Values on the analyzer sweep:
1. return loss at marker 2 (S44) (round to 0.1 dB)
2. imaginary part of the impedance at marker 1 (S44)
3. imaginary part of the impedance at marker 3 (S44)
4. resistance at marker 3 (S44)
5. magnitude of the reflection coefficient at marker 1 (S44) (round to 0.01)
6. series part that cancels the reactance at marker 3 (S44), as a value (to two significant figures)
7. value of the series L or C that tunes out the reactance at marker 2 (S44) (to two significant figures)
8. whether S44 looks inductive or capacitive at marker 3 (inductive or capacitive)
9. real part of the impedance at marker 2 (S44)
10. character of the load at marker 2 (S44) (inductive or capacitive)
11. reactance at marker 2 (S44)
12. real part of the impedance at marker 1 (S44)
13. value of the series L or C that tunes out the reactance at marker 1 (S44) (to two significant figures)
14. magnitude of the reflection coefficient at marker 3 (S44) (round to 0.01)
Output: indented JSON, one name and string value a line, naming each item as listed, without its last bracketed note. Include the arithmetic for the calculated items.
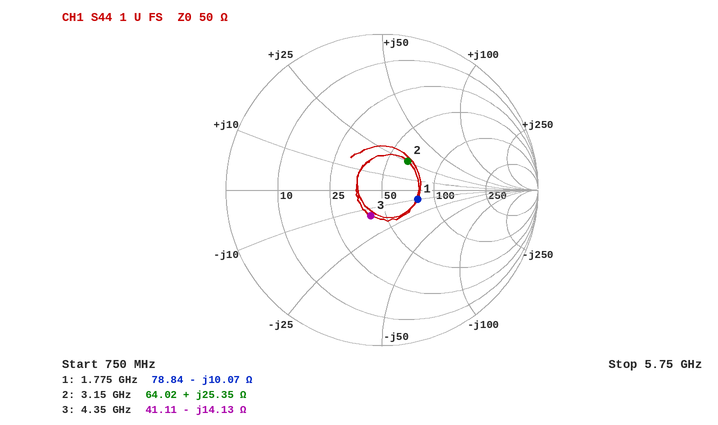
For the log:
{
  "return loss at marker 2 (S44)": "12.1 dB",
  "imaginary part of the impedance at marker 1": "-10.07 Ω",
  "imaginary part of the impedance at marker 3": "-14.13 Ω",
  "resistance at marker 3": "41.11 Ω",
  "magnitude of the reflection coefficient at marker 1 (S44)": "0.24",
  "series part that cancels the reactance at marker 3 (S44), as a value": "L = 14.13 Ω/(2π × 4.35 GHz) ≈ 517 pH, so 520 pH to two significant figures",
  "value of the series L or C that tunes out the reactance at marker 2 (S44)": "C = 1/(2π × 3.15 GHz × 25.35 Ω) ≈ 2.0 pF",
  "whether S44 looks inductive or capacitive at marker 3": "capacitive",
  "real part of the impedance at marker 2": "64.02 Ω",
  "character of the load at marker 2 (S44)": "inductive",
  "reactance at marker 2": "+25.35 Ω",
  "real part of the impedance at marker 1": "78.84 Ω",
  "value of the series L or C that tunes out the reactance at marker 1 (S44)": "L = 10.07 Ω/(2π × 1.775 GHz) ≈ 903 pH, so 900 pH to two significant figures",
  "magnitude of the reflection coefficient at marker 3 (S44)": "0.18"
}
